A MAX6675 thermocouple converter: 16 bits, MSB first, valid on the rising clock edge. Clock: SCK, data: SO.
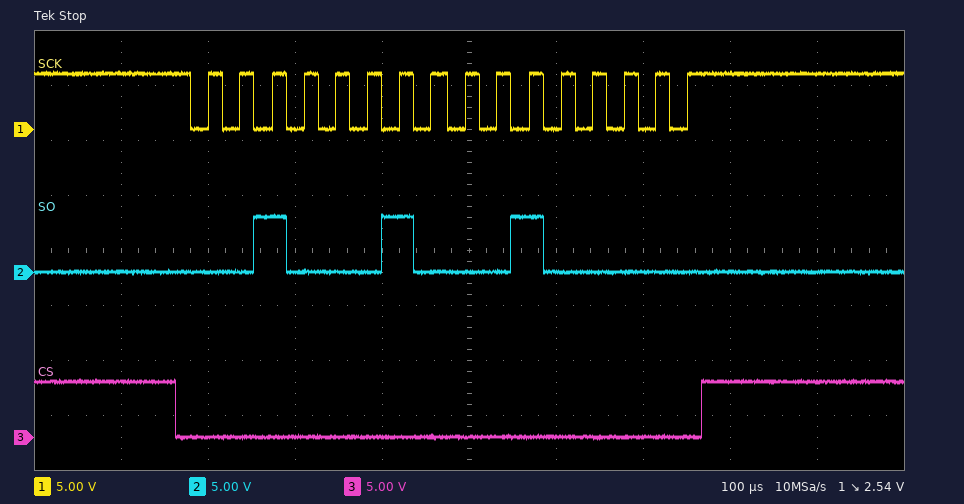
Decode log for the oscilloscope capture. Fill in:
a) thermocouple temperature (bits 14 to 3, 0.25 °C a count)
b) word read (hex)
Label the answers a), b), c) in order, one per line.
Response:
a) 273.00 °C
b) 0x2220
